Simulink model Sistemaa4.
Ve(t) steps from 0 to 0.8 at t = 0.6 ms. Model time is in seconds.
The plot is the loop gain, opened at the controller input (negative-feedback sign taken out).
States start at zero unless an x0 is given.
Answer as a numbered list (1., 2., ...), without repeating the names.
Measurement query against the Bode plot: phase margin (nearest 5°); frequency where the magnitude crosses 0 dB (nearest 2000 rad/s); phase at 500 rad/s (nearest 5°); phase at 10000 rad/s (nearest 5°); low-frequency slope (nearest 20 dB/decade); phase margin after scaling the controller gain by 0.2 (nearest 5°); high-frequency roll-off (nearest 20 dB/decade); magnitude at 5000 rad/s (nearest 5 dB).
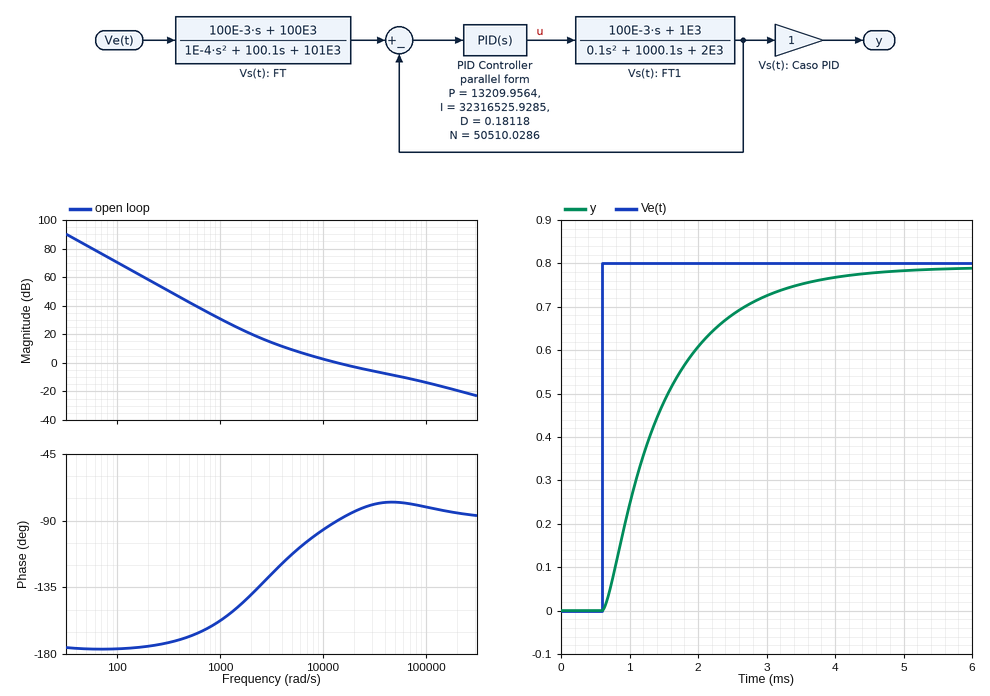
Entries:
1. 90°
2. 14000 rad/s
3. -170°
4. -95°
5. -40 dB/decade
6. 55°
7. -20 dB/decade
8. 10 dB
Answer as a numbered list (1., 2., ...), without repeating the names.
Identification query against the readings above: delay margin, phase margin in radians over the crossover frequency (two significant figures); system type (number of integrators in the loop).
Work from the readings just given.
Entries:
1. 0.00011 s
2. 2
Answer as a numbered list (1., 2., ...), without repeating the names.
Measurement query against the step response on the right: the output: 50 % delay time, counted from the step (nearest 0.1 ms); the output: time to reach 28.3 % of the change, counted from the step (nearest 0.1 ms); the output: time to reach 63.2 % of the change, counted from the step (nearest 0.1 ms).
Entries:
1. 0.7 ms
2. 0.4 ms
3. 1.0 ms
